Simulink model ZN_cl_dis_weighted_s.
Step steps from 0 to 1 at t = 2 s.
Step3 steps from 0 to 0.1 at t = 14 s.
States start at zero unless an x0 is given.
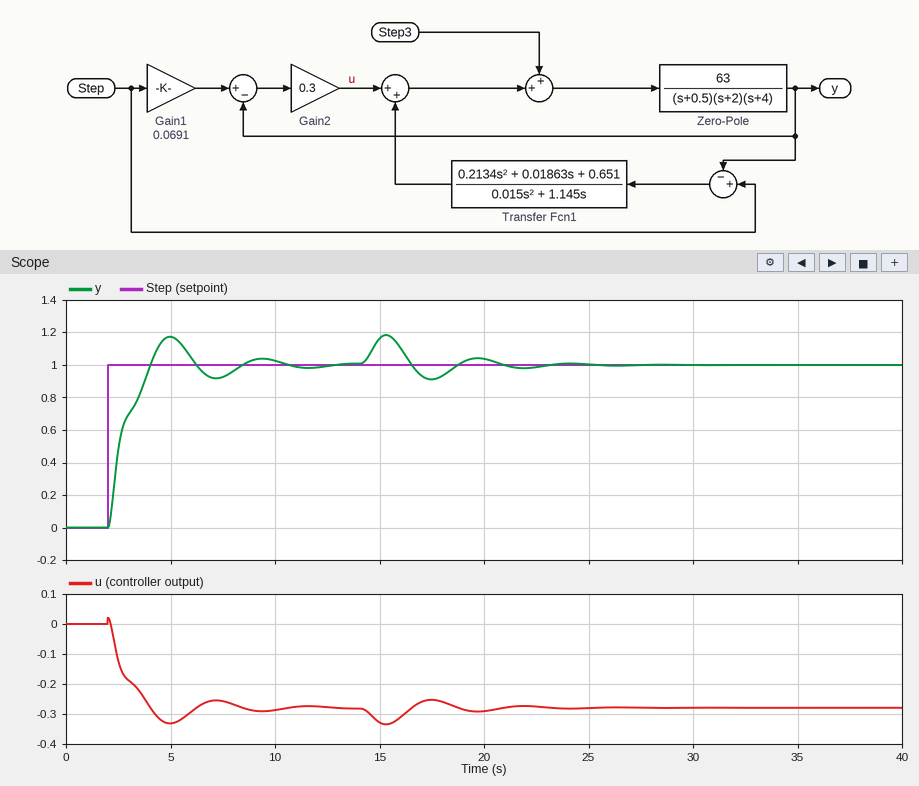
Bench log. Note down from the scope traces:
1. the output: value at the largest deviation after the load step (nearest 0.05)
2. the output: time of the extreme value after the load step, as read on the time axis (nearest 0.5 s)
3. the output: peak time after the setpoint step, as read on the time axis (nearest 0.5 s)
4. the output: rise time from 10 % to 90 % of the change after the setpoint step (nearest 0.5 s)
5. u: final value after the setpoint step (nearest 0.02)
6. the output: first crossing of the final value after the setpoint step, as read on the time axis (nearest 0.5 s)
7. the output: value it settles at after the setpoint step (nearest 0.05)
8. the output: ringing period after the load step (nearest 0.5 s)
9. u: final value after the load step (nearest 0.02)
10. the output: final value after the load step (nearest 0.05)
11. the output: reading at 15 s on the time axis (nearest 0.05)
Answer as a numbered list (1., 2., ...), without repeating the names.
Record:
1. 1.20
2. 15.5 s
3. 5.0 s
4. 1.5 s
5. -0.28
6. 4.0 s
7. 1.00
8. 4.5 s
9. -0.28
10. 1.00
11. 1.15
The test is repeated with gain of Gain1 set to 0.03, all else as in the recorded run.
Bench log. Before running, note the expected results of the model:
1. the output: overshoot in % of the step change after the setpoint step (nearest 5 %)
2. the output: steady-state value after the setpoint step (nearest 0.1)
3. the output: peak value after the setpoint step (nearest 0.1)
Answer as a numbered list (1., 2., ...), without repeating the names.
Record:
1. 20 %
2. 1.0
3. 1.2
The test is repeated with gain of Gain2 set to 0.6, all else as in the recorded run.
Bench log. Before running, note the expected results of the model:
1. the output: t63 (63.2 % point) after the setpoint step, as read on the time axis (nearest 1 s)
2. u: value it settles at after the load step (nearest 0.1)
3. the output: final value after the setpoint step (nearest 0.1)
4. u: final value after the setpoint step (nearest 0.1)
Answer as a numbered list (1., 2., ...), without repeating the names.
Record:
1. 4 s
2. -0.6
3. 1.0
4. -0.6
